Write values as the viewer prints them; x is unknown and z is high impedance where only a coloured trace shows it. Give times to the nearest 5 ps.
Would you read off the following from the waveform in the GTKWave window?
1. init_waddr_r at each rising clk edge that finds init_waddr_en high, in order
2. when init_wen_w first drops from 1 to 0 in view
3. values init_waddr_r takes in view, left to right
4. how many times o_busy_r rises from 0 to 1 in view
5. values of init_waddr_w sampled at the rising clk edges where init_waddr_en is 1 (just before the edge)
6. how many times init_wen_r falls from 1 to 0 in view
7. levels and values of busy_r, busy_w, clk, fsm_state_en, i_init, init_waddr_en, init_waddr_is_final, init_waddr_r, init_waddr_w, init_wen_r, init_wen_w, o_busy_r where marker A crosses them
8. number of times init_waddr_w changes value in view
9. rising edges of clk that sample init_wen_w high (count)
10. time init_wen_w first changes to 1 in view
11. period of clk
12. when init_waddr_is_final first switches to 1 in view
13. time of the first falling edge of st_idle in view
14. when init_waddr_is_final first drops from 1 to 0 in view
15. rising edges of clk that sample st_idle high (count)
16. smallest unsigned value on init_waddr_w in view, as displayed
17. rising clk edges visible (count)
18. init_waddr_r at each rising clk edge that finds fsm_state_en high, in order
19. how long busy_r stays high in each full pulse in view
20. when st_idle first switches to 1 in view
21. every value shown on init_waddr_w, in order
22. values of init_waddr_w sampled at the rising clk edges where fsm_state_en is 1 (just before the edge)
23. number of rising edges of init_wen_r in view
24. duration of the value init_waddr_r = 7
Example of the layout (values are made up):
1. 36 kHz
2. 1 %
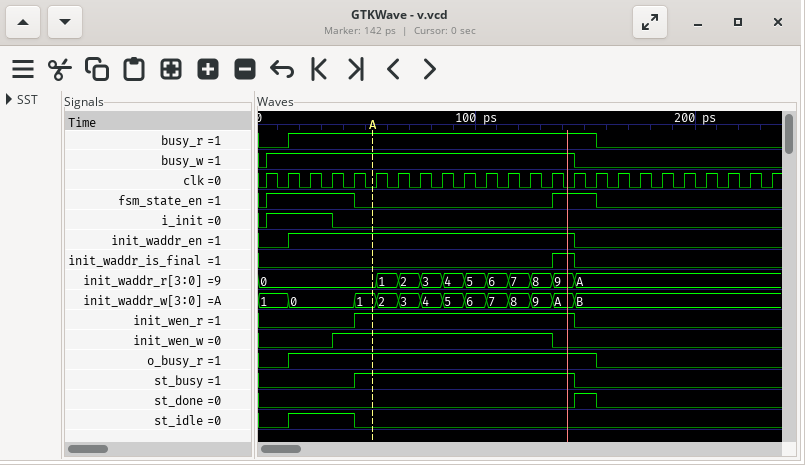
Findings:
1. 0, 0, 0, 0, 1, 2, 3, 4, 5, 6, 7, 8, 9
2. 135 ps
3. 0, 1, 2, 3, 4, 5, 6, 7, 8, 9, A
4. 1
5. 0, 0, 0, 1, 2, 3, 4, 5, 6, 7, 8, 9, A
6. 1
7. busy_r=1, busy_w=1, clk=0, fsm_state_en=0, i_init=0, init_waddr_en=1, init_waddr_is_final=0, init_waddr_r=0, init_waddr_w=1, init_wen_r=1, init_wen_w=1, o_busy_r=1
8. 12
9. 10
10. 35 ps
11. 10 ps
12. 135 ps
13. 45 ps
14. 145 ps
15. 3
16. 0
17. 24
18. 0, 0, 0, 0, 9, A
19. 140 ps
20. 15 ps
21. 1, 0, 1, 2, 3, 4, 5, 6, 7, 8, 9, A, B
22. 1, 0, 0, 0, A, B
23. 1
24. 10 ps
